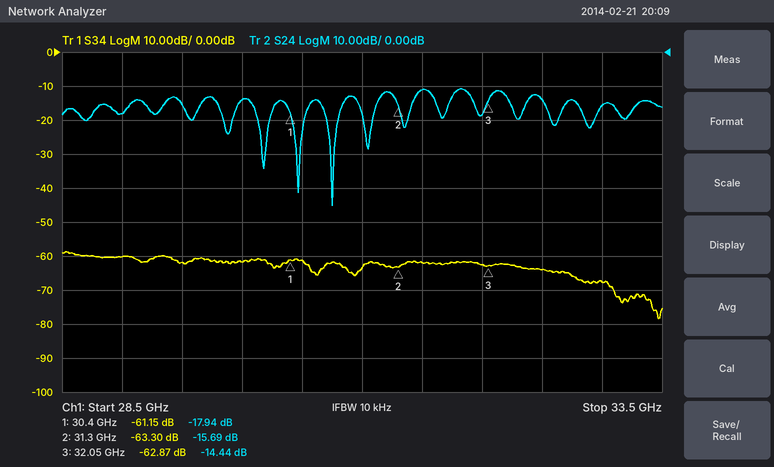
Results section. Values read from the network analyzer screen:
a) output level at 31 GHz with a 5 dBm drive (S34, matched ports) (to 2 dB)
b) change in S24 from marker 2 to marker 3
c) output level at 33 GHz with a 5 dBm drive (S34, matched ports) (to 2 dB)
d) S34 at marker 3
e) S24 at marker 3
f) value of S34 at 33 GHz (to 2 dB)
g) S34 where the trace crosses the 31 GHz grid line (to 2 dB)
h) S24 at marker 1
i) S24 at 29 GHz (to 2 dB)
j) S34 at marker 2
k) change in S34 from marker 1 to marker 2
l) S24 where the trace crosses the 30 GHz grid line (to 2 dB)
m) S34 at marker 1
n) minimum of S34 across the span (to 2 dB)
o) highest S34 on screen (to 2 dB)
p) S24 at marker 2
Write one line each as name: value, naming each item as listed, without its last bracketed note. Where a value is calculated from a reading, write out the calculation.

output level at 31 GHz with a 5 dBm drive (S34, matched ports): 5 dBm + (-64 dB) = -58 dBm
change in S24 from marker 2 to marker 3: -14.44 − (-15.69) = 1.25 dB
output level at 33 GHz with a 5 dBm drive (S34, matched ports): 5 dBm + (-68 dB) = -62 dBm
S34 at marker 3: -62.87 dB
S24 at marker 3: -14.44 dB
value of S34 at 33 GHz: -68 dB
S34 where the trace crosses the 31 GHz grid line: -64 dB
S24 at marker 1: -17.94 dB
S24 at 29 GHz: -18 dB
S34 at marker 2: -63.30 dB
change in S34 from marker 1 to marker 2: -63.3 − (-61.15) = -2.15 dB
S24 where the trace crosses the 30 GHz grid line: -14 dB
S34 at marker 1: -61.15 dB
minimum of S34 across the span: -78 dB
highest S34 on screen: -58 dB
S24 at marker 2: -15.69 dB
